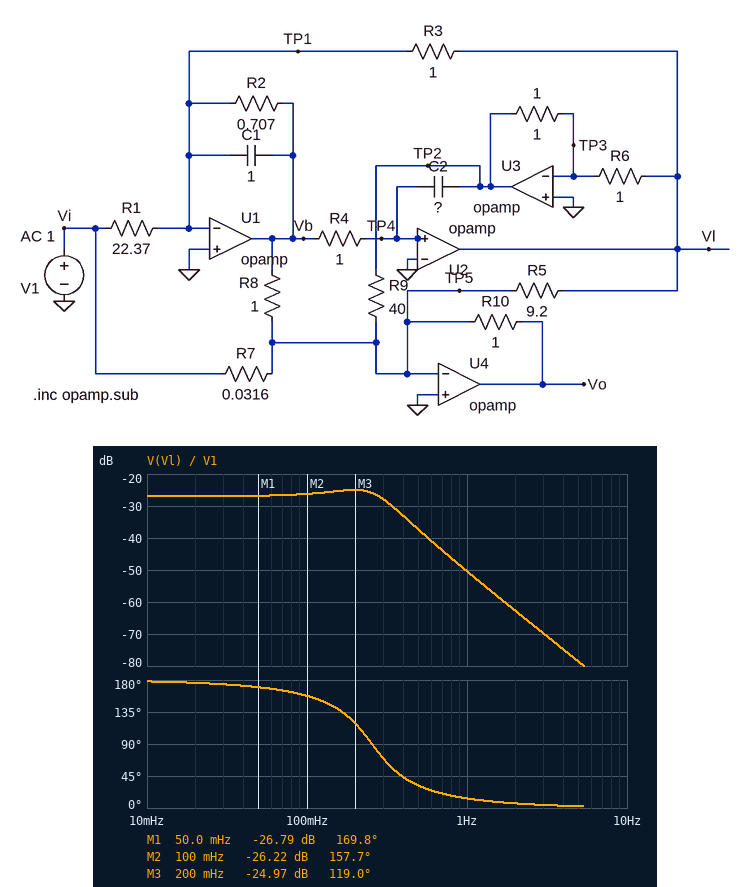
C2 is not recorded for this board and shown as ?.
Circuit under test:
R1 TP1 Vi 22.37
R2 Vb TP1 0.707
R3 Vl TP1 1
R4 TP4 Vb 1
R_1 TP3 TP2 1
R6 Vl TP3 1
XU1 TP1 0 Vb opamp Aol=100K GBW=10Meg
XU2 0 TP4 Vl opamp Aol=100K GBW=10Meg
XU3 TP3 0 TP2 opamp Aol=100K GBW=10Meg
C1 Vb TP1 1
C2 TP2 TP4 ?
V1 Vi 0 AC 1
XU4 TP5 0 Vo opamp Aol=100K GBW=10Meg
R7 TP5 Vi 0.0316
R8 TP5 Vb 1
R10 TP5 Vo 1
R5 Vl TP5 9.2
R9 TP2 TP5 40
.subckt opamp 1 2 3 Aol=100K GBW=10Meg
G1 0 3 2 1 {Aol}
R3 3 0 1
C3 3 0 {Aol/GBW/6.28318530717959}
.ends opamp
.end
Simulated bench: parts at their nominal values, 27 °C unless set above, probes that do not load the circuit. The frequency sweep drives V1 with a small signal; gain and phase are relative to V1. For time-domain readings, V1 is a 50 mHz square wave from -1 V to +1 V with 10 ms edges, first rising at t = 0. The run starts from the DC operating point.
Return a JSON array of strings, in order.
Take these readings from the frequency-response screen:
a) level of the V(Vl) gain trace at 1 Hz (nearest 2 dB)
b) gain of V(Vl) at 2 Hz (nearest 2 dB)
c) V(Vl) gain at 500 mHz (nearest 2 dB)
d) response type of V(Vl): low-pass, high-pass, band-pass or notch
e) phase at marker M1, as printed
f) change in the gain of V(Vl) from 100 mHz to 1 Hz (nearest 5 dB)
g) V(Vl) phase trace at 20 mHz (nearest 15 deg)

["-50 dB", "-62 dB", "-38 dB", "low-pass", "169.8 deg", "-25 dB", "180 deg"]
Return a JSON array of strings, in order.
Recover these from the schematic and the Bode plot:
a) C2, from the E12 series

["390 mF"]
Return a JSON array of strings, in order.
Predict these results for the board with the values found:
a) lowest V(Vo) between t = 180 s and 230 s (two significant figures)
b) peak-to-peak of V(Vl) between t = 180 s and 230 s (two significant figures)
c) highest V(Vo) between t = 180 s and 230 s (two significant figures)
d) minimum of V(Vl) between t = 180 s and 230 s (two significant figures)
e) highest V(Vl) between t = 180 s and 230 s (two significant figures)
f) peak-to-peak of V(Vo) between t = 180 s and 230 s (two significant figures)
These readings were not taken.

["-32 V", "130 mV", "32 V", "-64 mV", "64 mV", "63 V"]
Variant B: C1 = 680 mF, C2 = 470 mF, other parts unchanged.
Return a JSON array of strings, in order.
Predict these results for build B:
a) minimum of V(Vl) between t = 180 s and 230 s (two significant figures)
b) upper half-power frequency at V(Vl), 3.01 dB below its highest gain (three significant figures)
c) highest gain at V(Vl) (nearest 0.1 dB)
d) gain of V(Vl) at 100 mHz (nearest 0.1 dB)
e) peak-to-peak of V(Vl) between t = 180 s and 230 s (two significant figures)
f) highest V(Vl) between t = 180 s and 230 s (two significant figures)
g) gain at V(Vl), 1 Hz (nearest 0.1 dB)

["-54 mV", "316 mHz", "-26.6 dB", "-26.7 dB", "110 mV", "54 mV", "-48.8 dB"]
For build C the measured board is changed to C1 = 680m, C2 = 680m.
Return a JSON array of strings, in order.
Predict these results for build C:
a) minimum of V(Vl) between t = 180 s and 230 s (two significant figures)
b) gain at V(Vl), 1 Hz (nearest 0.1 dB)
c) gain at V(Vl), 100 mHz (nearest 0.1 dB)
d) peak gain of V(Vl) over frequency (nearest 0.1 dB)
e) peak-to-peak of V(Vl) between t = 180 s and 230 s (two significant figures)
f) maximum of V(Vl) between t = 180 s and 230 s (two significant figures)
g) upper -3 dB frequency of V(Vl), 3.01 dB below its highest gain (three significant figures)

["-49 mV", "-52.2 dB", "-27.1 dB", "-27.0 dB", "97 mV", "49 mV", "234 mHz"]
